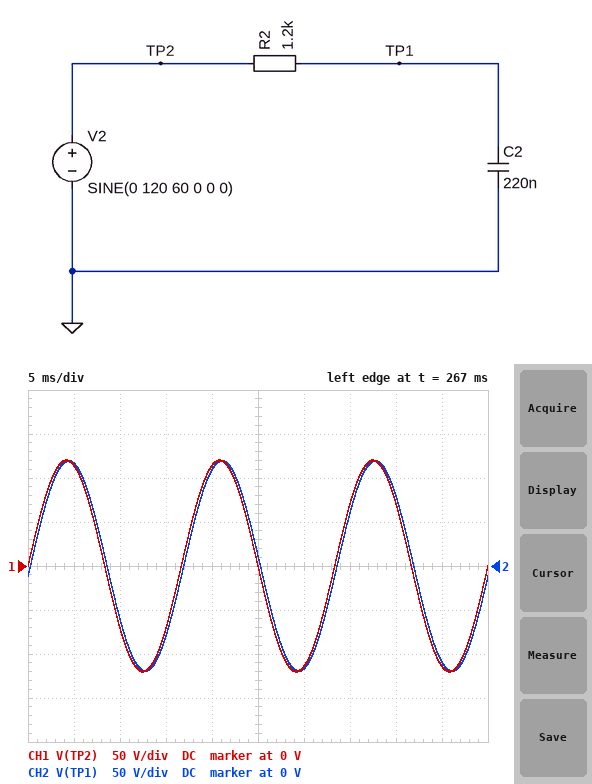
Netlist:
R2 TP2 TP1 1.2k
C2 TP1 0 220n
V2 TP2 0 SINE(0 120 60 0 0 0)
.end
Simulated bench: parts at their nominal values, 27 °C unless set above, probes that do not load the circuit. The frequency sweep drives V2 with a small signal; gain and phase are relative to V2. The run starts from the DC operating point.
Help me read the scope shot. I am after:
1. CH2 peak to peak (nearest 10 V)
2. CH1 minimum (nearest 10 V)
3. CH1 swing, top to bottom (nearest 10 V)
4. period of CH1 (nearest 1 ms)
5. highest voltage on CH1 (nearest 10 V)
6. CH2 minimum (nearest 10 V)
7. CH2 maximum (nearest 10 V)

240 V
-120 V
240 V
17 ms
120 V
-120 V
120 V
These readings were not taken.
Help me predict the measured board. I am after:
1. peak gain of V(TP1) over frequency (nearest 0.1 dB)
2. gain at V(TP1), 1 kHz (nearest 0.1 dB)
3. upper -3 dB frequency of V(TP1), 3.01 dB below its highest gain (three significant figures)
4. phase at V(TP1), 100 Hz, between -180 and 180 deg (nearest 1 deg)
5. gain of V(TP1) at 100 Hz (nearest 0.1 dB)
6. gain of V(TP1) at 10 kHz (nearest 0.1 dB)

0 dB
-5.7 dB
603 Hz
-9 deg
-0.1 dB
-24.4 dB
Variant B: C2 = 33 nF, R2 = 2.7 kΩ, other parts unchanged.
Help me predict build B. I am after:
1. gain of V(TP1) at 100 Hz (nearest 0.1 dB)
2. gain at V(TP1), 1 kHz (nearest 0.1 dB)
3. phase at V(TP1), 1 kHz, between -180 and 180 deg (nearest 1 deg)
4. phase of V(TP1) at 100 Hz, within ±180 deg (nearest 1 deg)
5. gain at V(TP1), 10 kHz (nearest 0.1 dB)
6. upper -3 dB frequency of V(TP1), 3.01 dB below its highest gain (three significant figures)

0 dB
-1.2 dB
-29 deg
-3 deg
-15.1 dB
1.79 kHz
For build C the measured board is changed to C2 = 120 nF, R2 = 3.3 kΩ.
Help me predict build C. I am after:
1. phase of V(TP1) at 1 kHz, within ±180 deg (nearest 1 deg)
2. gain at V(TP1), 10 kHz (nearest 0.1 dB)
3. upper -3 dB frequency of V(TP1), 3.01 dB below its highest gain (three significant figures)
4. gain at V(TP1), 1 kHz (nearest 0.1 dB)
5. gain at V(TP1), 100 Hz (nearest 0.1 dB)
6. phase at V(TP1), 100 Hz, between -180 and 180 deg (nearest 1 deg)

-68 deg
-27.9 dB
402 Hz
-8.6 dB
-0.3 dB
-14 deg
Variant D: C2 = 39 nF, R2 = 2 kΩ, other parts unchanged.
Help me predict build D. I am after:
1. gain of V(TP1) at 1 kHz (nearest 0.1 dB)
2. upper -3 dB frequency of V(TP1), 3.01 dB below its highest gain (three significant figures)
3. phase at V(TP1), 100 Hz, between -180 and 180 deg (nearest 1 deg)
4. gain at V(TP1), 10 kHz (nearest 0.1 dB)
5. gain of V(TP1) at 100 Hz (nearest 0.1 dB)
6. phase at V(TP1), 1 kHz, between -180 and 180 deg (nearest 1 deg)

-0.9 dB
2.04 kHz
-3 deg
-14.0 dB
0 dB
-26 deg
